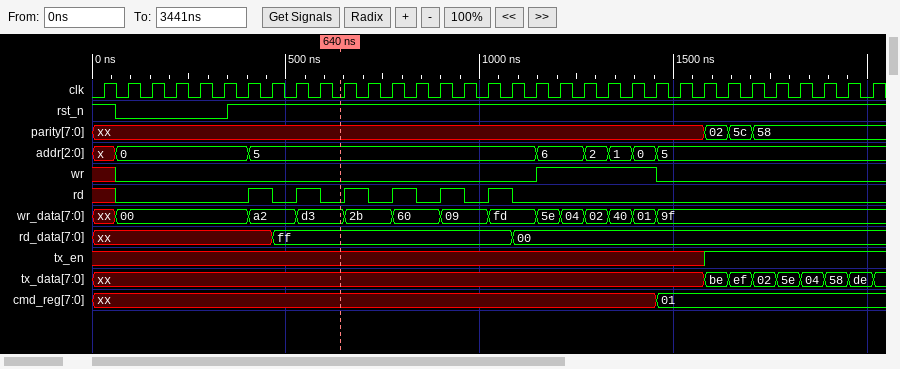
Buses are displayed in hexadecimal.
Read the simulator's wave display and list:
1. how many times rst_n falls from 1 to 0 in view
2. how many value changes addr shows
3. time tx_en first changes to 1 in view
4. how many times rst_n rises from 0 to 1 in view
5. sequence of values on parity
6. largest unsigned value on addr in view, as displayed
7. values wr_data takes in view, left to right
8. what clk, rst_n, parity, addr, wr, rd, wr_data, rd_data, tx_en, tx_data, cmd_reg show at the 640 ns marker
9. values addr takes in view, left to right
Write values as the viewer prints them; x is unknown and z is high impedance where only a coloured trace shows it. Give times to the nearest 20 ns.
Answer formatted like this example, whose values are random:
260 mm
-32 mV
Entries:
1
7
1580 ns
1
xx, 02, 5c, 58
6
xx, 00, a2, d3, 2b, 60, 09, fd, 5e, 04, 02, 40, 01, 9f
clk=0, rst_n=1, parity=xx, addr=5, wr=0, rd=0, wr_data=d3, rd_data=ff, tx_en=x, tx_data=xx, cmd_reg=xx
x, 0, 5, 6, 2, 1, 0, 5
